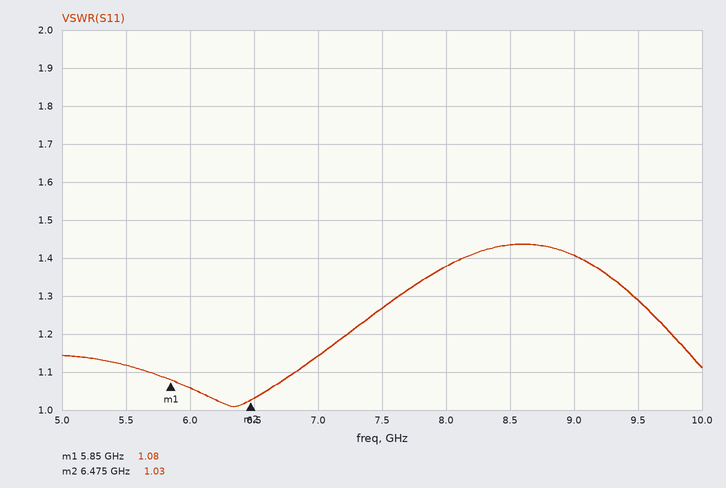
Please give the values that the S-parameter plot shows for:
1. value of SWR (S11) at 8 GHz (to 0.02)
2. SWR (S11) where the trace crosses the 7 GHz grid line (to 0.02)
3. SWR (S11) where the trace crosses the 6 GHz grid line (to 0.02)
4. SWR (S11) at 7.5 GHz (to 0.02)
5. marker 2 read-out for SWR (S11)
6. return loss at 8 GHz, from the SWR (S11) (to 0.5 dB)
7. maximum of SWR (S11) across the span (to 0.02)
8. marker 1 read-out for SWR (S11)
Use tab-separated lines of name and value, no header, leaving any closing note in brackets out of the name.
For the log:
value of SWR (S11) at 8 GHz	1.38
SWR (S11) where the trace crosses the 7 GHz grid line	1.14
SWR (S11) where the trace crosses the 6 GHz grid line	1.06
SWR (S11) at 7.5 GHz	1.26
marker 2 read-out for SWR	1.03
return loss at 8 GHz, from the SWR (S11)	16.0 dB
maximum of SWR (S11) across the span	1.44
marker 1 read-out for SWR	1.08
